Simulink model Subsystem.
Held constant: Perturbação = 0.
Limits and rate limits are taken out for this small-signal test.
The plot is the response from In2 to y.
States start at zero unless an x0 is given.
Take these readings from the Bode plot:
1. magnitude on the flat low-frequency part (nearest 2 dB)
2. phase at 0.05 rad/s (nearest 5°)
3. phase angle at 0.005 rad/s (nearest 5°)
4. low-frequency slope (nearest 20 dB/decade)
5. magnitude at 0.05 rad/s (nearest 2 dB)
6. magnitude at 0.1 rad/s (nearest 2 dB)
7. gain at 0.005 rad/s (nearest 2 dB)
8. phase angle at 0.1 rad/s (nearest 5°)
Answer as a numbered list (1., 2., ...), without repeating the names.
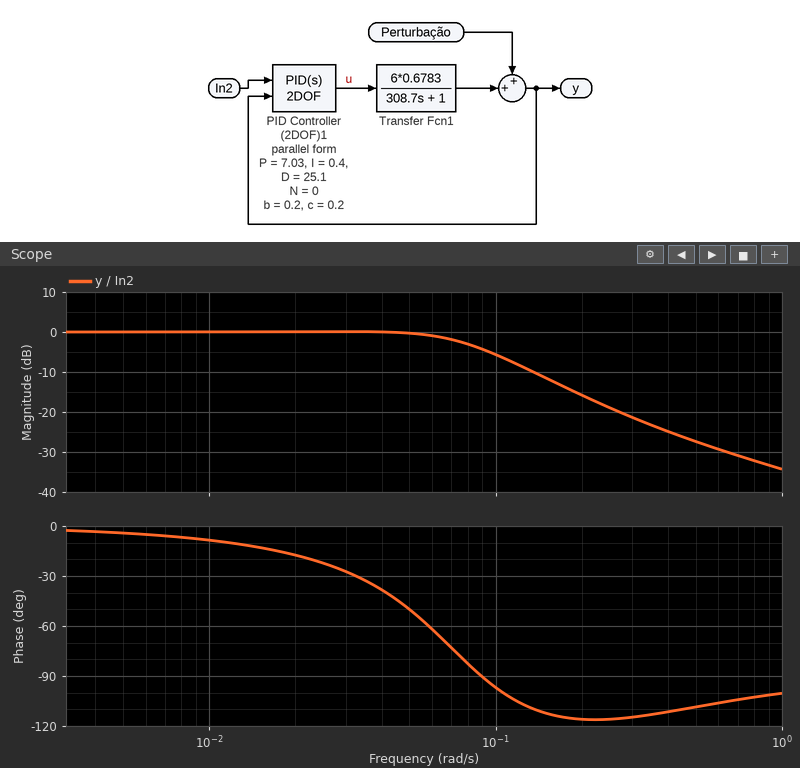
1. 0 dB
2. -50°
3. -5°
4. 0 dB/decade
5. 0 dB
6. -6 dB
7. 0 dB
8. -95°
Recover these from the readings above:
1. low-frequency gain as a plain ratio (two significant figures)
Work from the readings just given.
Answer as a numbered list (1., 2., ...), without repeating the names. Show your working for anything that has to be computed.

1. 10^(0 / 20) = 1.0
